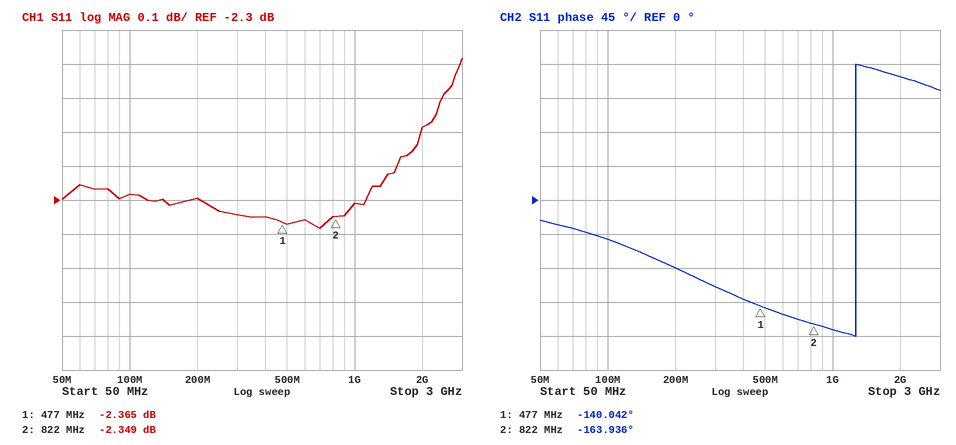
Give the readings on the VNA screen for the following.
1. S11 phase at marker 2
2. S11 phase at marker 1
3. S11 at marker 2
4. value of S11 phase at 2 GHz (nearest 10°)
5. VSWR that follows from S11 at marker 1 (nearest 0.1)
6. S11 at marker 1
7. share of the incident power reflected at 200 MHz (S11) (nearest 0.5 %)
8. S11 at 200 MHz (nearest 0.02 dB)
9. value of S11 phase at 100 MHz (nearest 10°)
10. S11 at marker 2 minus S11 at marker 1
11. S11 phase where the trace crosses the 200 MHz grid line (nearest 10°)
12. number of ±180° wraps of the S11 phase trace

-163.936°
-140.042°
-2.349 dB
160°
7.4
-2.365 dB
59.0 %
-2.30 dB
-50°
0.016 dB
-90°
1
